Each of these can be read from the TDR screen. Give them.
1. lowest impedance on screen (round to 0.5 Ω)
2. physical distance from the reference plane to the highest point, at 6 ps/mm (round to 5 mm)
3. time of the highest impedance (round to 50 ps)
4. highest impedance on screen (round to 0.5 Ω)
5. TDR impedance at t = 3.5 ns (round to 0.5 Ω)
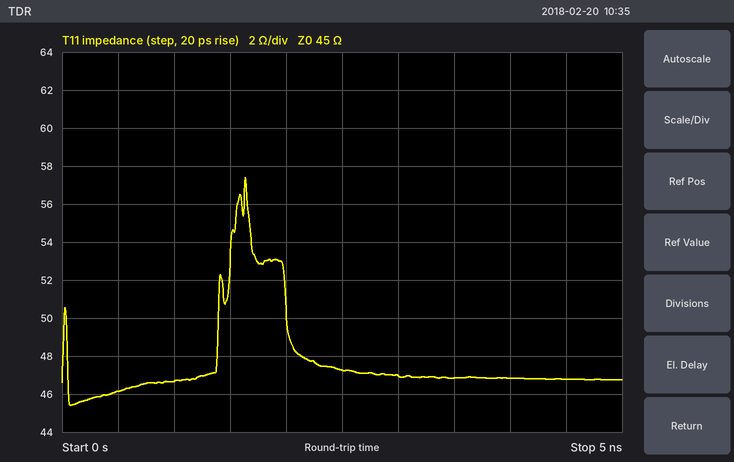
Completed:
45.5 Ω
135 mm
1.65 ns
57.5 Ω
47.0 Ω
